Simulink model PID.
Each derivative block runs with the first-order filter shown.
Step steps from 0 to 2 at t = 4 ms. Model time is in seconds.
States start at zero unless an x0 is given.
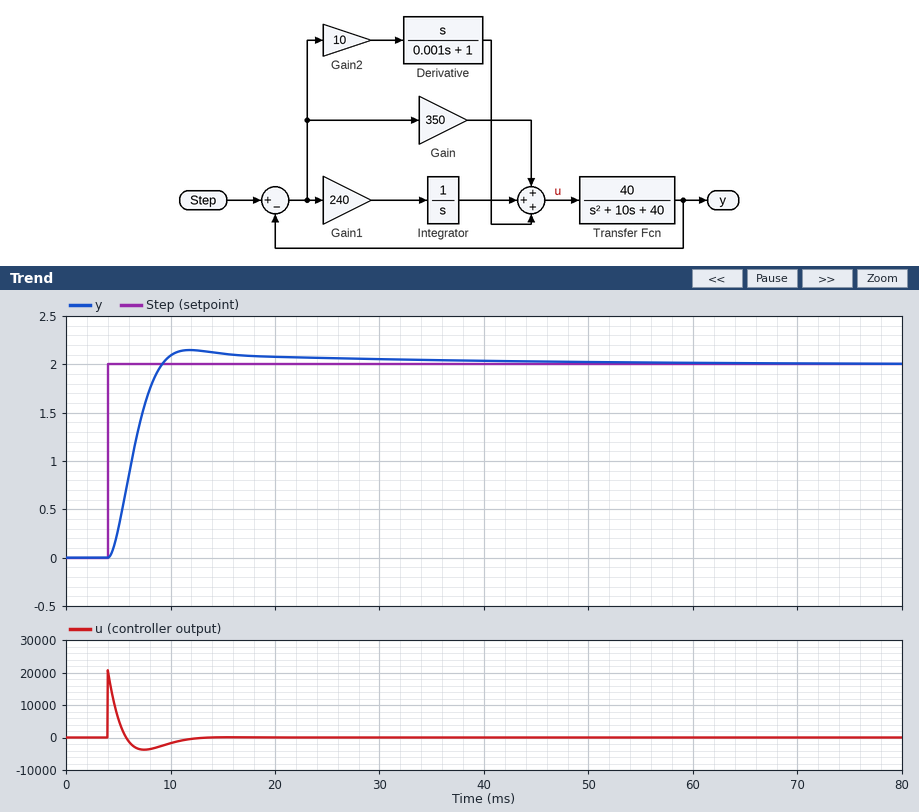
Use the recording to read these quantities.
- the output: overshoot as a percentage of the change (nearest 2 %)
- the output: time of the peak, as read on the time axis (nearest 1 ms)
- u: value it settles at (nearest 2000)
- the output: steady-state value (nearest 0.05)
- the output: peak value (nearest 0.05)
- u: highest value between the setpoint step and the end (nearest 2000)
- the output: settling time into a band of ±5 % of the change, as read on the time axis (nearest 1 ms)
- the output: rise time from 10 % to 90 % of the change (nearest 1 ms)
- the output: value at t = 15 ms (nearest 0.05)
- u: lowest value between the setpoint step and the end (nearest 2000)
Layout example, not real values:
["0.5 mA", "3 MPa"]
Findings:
["8 %", "12 ms", "0", "2.00", "2.15", "20000", "16 ms", "3 ms", "2.10", "-4000"]
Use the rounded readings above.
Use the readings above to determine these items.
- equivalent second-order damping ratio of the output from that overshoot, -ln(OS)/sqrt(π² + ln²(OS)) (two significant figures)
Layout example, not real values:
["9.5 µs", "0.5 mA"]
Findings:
["0.63"]
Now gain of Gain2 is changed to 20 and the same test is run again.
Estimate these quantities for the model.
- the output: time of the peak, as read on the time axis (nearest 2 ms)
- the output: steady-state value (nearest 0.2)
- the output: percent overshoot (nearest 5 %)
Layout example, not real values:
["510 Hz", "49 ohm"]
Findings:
["8 ms", "2.0", "15 %"]
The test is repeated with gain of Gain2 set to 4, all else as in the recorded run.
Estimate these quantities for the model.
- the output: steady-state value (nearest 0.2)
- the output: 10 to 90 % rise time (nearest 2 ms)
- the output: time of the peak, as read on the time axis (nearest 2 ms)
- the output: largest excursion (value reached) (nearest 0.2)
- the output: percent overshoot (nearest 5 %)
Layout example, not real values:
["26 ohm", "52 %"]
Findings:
["2.0", "6 ms", "22 ms", "2.4", "20 %"]
